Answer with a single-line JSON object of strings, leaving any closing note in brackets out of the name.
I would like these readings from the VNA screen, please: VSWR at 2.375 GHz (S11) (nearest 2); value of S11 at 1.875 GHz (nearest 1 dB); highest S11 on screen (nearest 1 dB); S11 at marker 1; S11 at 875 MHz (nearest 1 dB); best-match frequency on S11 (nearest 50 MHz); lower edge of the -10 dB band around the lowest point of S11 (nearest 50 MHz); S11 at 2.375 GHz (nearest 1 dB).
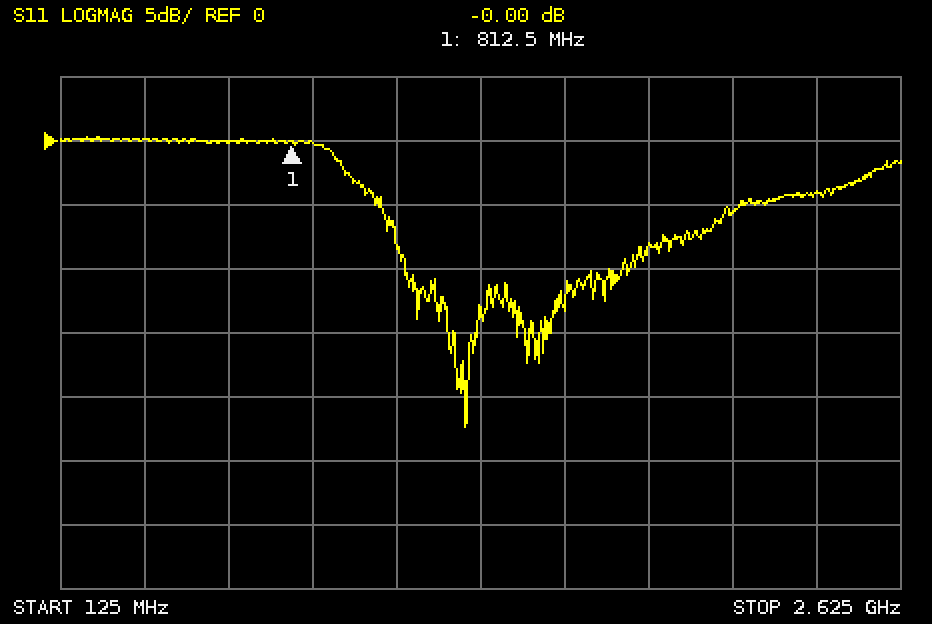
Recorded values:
{"VSWR at 2.375 GHz (S11)": "4", "value of S11 at 1.875 GHz": "-8 dB", "highest S11 on screen": "0 dB", "S11 at marker 1": "-0.00 dB", "S11 at 875 MHz": "0 dB", "best-match frequency on S11": "1.35 GHz", "lower edge of the -10 dB band around the lowest point of S11": "1.15 GHz", "S11 at 2.375 GHz": "-4 dB"}
